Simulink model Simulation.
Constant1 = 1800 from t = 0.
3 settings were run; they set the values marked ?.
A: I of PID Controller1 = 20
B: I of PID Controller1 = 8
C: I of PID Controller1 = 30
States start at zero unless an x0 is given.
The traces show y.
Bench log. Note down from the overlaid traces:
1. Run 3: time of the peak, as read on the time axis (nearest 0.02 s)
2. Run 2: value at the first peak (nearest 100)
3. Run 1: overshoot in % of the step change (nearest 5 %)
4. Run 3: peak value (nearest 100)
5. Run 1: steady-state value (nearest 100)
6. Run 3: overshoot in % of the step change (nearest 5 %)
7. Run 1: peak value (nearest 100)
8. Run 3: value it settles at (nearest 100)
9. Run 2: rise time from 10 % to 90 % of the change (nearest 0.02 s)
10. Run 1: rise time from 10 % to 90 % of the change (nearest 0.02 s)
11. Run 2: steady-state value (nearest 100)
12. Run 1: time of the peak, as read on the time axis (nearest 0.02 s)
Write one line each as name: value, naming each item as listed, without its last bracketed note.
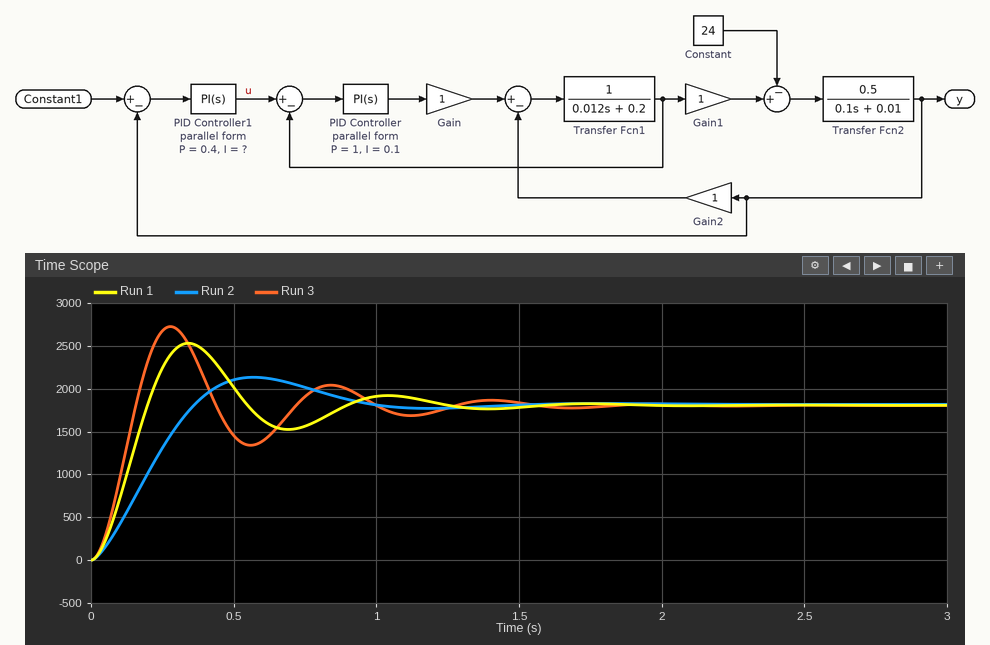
Run 3: time of the peak, as read on the time axis: 0.28 s
Run 2: value at the first peak: 2100
Run 1: overshoot in % of the step change: 40 %
Run 3: peak value: 2700
Run 1: steady-state value: 1800
Run 3: overshoot in % of the step change: 50 %
Run 1: peak value: 2500
Run 3: value it settles at: 1800
Run 2: rise time from 10 % to 90 % of the change: 0.26 s
Run 1: rise time from 10 % to 90 % of the change: 0.14 s
Run 2: steady-state value: 1800
Run 1: time of the peak, as read on the time axis: 0.34 s
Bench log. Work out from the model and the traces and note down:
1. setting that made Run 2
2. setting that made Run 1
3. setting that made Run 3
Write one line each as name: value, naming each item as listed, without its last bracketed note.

setting that made Run 2: B
setting that made Run 1: A
setting that made Run 3: C
